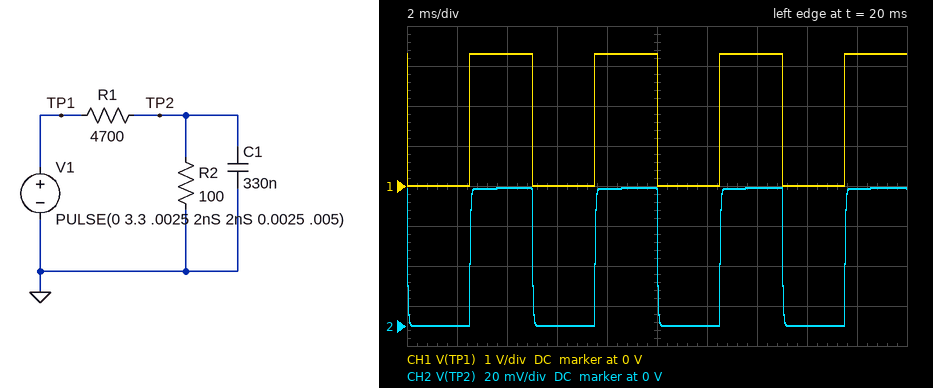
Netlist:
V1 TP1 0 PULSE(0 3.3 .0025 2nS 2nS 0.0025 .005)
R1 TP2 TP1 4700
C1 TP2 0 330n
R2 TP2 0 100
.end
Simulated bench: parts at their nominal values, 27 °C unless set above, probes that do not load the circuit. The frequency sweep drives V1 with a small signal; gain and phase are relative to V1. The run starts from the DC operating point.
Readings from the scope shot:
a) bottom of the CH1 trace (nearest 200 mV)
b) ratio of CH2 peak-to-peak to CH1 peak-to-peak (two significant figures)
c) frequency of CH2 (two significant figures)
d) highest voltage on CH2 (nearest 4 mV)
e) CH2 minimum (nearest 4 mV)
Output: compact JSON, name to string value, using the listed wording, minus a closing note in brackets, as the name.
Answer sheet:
{"bottom of the CH1 trace": "0 V", "ratio of CH2 peak-to-peak to CH1 peak-to-peak": "0.021", "frequency of CH2": "200 Hz", "highest voltage on CH2": "68 mV", "CH2 minimum": "0 V"}
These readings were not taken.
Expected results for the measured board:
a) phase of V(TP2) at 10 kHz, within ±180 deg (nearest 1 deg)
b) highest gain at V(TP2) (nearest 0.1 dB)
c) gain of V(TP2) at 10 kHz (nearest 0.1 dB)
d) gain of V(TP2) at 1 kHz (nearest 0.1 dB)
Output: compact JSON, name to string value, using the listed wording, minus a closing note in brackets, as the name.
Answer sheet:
{"phase of V(TP2) at 10 kHz, within ±180 deg": "-64 deg", "highest gain at V(TP2)": "-33.6 dB", "gain of V(TP2) at 10 kHz": "-40.7 dB", "gain of V(TP2) at 1 kHz": "-33.8 dB"}
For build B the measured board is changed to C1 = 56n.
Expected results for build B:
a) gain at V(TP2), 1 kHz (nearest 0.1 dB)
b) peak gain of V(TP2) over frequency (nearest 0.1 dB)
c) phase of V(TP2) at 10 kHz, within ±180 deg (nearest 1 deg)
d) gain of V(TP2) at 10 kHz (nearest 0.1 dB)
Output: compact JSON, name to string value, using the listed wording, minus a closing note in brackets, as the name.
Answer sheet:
{"gain at V(TP2), 1 kHz": "-33.6 dB", "peak gain of V(TP2) over frequency": "-33.6 dB", "phase of V(TP2) at 10 kHz, within ±180 deg": "-19 deg", "gain of V(TP2) at 10 kHz": "-34.1 dB"}
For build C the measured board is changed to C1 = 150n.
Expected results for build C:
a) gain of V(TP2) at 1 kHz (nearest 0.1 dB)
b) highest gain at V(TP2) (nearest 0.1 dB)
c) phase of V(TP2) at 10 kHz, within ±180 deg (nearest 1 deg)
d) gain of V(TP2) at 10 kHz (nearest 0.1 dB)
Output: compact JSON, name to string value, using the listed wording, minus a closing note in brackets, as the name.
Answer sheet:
{"gain of V(TP2) at 1 kHz": "-33.7 dB", "highest gain at V(TP2)": "-33.6 dB", "phase of V(TP2) at 10 kHz, within ±180 deg": "-43 deg", "gain of V(TP2) at 10 kHz": "-36.3 dB"}
